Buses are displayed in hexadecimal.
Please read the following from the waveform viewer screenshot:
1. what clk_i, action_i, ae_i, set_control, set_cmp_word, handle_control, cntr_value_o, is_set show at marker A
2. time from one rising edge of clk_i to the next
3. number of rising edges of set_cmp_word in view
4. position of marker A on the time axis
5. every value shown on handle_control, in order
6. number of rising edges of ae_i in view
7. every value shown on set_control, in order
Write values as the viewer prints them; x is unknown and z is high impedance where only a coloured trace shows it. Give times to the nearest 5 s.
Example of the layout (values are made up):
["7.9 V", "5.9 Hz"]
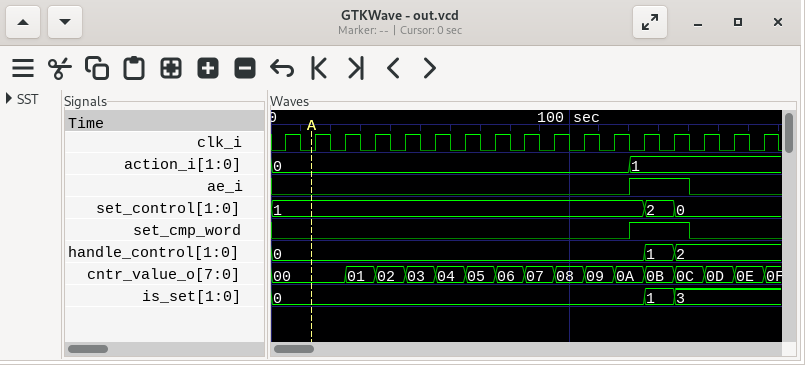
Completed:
["clk_i=0, action_i=0, ae_i=0, set_control=1, set_cmp_word=0, handle_control=0, cntr_value_o=00, is_set=0", "10 s", "1", "15 s", "0, 1, 2", "1", "1, 2, 0"]
